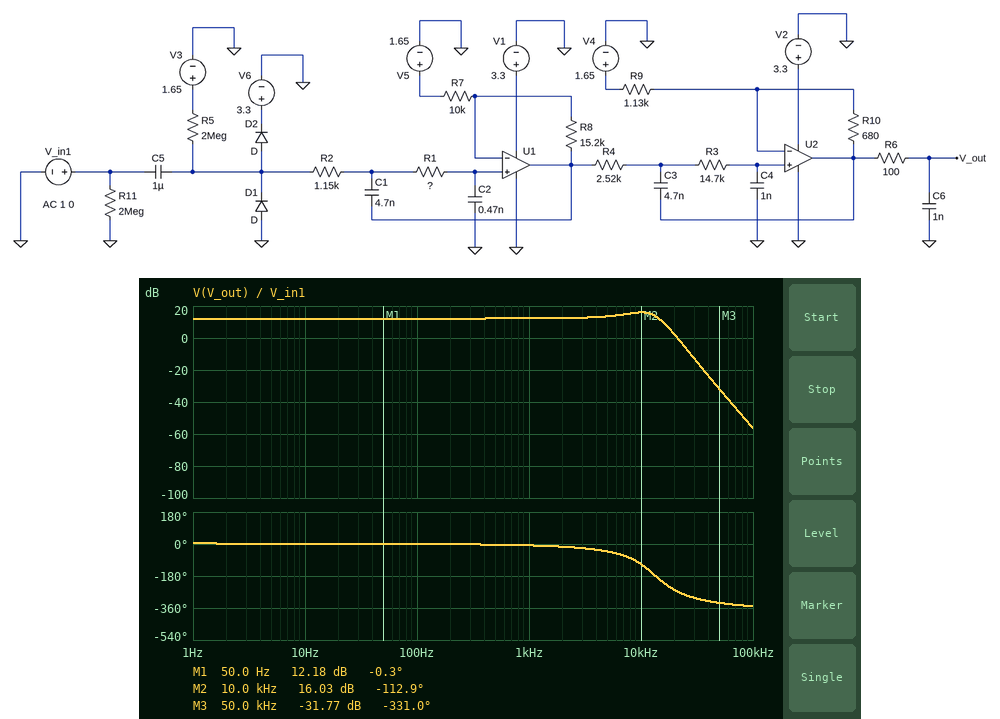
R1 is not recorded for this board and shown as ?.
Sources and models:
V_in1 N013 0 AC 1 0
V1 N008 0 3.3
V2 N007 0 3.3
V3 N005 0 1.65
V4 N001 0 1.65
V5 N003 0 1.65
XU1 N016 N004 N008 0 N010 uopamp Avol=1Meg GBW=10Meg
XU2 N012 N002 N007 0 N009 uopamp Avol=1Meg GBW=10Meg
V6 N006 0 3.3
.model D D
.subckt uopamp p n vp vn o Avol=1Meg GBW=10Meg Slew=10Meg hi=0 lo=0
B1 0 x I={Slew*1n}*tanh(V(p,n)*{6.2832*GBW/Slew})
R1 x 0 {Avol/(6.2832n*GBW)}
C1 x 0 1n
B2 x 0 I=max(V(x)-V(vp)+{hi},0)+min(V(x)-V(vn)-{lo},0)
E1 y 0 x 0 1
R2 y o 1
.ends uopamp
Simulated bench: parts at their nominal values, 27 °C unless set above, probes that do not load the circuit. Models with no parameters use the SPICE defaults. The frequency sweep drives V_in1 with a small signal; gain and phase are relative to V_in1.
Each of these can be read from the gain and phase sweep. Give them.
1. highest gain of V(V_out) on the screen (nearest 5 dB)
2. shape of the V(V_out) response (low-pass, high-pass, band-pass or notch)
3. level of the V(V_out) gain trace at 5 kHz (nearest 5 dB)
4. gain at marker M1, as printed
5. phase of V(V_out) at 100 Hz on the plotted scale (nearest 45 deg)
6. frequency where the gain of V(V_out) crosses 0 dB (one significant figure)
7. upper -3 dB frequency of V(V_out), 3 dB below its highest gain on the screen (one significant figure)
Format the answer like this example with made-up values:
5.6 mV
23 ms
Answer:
15 dB
low-pass
15 dB
12.18 dB
0 deg
20 kHz
10 kHz
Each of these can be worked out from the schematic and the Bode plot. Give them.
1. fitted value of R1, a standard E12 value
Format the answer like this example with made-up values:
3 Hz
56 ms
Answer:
39 kΩ
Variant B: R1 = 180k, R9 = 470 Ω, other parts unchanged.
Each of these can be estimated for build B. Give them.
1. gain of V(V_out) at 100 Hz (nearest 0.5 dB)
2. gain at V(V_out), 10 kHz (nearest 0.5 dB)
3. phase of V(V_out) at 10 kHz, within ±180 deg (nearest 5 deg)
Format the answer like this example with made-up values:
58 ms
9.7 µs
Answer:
16.0 dB
12.0 dB
-100 deg
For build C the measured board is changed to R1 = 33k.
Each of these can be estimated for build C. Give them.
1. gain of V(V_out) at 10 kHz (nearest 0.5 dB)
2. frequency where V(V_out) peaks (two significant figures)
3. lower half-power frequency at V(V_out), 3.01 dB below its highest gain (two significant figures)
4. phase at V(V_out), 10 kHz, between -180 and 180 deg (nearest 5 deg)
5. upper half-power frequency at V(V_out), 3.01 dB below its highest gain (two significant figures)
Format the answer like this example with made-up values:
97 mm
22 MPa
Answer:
17.0 dB
11 kHz
5.4 kHz
-100 deg
15 kHz
